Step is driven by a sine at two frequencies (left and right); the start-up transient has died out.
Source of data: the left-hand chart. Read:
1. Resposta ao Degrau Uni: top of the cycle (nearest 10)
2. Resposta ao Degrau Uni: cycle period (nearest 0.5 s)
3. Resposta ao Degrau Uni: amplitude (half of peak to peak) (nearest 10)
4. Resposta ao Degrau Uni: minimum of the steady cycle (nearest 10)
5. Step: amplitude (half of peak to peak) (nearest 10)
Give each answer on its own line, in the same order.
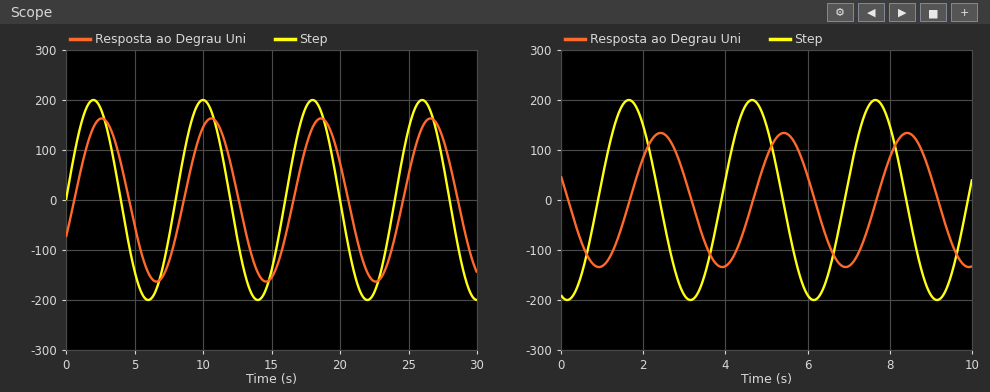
160
8.0 s
160
-160
200
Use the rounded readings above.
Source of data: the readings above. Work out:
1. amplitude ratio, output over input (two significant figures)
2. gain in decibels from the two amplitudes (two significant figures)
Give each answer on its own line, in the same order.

0.80
-1.9 dB
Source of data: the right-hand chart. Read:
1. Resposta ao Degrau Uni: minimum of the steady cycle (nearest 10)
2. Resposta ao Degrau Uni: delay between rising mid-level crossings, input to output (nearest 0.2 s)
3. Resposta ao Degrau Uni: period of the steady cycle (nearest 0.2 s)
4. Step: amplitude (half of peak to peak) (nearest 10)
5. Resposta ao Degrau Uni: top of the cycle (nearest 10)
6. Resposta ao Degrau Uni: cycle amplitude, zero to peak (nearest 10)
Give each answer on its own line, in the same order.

-130
0.8 s
3.0 s
200
130
130
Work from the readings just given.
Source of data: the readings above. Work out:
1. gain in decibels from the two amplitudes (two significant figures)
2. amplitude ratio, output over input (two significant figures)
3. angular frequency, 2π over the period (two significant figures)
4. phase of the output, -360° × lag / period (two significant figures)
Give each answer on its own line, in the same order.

-3.7 dB
0.65
2.1 rad/s
-96°
